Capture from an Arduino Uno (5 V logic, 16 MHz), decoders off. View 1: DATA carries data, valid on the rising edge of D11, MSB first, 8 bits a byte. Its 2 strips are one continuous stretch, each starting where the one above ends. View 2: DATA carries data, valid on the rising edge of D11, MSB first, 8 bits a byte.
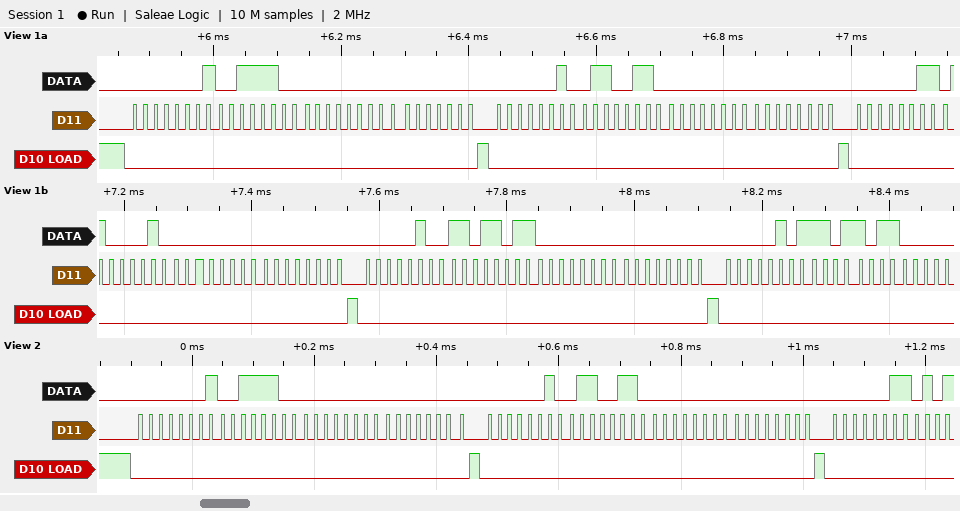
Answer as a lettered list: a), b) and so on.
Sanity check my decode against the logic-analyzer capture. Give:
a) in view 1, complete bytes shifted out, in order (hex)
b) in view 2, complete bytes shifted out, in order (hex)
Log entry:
a) 0x01 0x3C 0x00 0x00 0x02 0x66 0x00 0x00 0x03 0x42 0x00 0x00 0x04 0xDB 0x00 0x00 0x05 0xDB
b) 01 3C 00 00 02 66 00 00 03
